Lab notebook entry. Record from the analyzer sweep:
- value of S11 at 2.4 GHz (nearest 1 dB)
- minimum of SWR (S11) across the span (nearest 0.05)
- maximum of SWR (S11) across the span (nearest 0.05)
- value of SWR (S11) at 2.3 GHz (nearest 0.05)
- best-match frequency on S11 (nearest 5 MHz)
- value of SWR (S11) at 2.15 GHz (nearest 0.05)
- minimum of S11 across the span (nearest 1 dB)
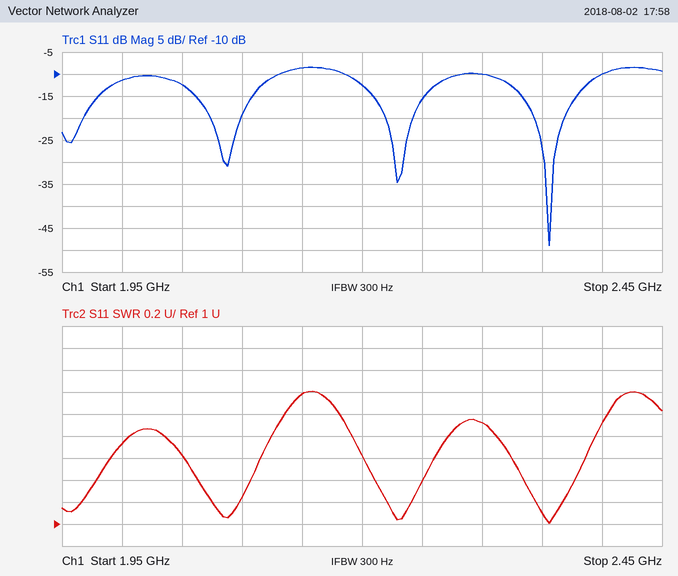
-10 dB
1.00
2.20
1.90
2.355 GHz
2.20
-49 dB
